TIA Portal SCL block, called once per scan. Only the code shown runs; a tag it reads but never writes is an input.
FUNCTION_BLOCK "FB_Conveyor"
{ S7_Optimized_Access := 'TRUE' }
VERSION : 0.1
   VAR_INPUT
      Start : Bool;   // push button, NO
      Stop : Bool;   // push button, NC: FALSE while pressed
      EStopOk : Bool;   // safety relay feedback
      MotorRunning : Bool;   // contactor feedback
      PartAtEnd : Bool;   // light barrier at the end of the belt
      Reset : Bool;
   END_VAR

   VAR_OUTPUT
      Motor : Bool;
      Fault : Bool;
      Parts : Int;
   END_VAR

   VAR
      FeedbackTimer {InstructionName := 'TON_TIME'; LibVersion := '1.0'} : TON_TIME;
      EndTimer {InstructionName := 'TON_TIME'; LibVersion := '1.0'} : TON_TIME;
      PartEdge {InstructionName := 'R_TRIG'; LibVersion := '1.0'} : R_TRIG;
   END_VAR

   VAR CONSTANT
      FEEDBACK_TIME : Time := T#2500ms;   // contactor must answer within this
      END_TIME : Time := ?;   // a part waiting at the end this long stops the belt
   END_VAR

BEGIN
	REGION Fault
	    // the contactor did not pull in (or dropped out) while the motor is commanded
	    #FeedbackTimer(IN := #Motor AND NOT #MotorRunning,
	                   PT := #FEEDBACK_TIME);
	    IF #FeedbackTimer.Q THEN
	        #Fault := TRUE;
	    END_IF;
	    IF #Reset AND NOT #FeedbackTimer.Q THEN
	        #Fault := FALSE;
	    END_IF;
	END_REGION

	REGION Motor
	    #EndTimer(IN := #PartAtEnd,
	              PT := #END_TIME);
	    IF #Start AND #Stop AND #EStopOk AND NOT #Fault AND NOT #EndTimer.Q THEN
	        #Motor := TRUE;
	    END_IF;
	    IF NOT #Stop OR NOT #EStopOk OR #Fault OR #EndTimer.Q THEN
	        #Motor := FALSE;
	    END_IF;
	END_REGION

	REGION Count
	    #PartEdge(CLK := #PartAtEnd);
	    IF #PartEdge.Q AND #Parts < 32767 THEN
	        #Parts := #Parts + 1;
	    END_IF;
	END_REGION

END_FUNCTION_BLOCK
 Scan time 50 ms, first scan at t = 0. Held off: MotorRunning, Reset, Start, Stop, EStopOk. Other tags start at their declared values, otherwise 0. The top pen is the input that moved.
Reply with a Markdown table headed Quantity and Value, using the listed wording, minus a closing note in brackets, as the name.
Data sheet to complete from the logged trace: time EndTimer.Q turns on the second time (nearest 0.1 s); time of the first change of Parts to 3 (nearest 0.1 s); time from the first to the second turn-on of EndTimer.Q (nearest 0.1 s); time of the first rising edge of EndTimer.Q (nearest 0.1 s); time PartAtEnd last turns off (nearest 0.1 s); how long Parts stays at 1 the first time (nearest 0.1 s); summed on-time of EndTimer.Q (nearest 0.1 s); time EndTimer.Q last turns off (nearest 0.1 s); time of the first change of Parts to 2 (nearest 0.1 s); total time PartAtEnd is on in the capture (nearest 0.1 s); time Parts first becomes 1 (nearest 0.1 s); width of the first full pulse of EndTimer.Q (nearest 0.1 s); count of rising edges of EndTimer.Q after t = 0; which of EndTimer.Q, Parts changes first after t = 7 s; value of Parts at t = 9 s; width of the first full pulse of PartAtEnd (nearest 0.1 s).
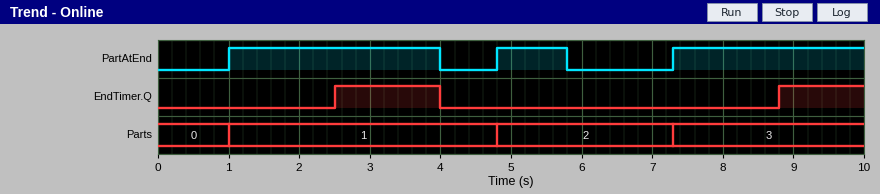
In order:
| Quantity | Value |
|---|---|
| time EndTimer.Q turns on the second time | 8.8 s |
| time of the first change of Parts to 3 | 7.3 s |
| time from the first to the second turn-on of EndTimer.Q | 6.3 s |
| time of the first rising edge of EndTimer.Q | 2.5 s |
| time PartAtEnd last turns off | 5.8 s |
| how long Parts stays at 1 the first time | 3.8 s |
| summed on-time of EndTimer.Q | 2.7 s |
| time EndTimer.Q last turns off | 4.0 s |
| time of the first change of Parts to 2 | 4.8 s |
| total time PartAtEnd is on in the capture | 6.7 s |
| time Parts first becomes 1 | 1.0 s |
| width of the first full pulse of EndTimer.Q | 1.5 s |
| count of rising edges of EndTimer.Q after t = 0 | 2 |
| which of EndTimer.Q, Parts changes first after t = 7 s | Parts |
| value of Parts at t = 9 s | 3 |
| width of the first full pulse of PartAtEnd | 3.0 s |
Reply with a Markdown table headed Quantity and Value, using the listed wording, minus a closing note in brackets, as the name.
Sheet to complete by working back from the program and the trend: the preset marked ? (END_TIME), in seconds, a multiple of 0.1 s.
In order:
| Quantity | Value |
|---|---|
| the preset marked ? (END_TIME), in seconds, a multiple of 0.1 s | 1.5 s |
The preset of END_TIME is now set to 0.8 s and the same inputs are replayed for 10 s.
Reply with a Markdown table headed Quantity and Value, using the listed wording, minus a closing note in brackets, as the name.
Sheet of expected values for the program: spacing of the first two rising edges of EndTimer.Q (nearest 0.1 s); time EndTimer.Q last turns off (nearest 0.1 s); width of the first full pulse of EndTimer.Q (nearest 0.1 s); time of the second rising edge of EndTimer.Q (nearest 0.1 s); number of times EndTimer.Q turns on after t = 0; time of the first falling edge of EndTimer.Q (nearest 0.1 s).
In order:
| Quantity | Value |
|---|---|
| spacing of the first two rising edges of EndTimer.Q | 3.8 s |
| time EndTimer.Q last turns off | 5.8 s |
| width of the first full pulse of EndTimer.Q | 2.2 s |
| time of the second rising edge of EndTimer.Q | 5.6 s |
| number of times EndTimer.Q turns on after t = 0 | 3 |
| time of the first falling edge of EndTimer.Q | 4.0 s |
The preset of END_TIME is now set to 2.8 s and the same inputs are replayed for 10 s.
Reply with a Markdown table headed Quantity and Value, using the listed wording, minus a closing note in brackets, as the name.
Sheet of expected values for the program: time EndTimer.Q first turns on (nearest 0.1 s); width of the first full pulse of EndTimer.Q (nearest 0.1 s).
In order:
| Quantity | Value |
|---|---|
| time EndTimer.Q first turns on | 3.8 s |
| width of the first full pulse of EndTimer.Q | 0.2 s |
